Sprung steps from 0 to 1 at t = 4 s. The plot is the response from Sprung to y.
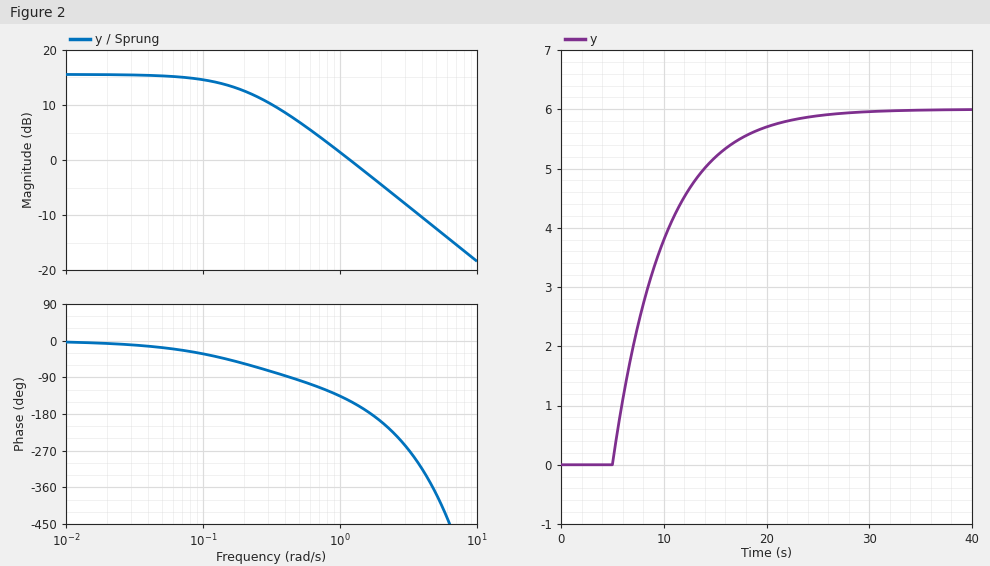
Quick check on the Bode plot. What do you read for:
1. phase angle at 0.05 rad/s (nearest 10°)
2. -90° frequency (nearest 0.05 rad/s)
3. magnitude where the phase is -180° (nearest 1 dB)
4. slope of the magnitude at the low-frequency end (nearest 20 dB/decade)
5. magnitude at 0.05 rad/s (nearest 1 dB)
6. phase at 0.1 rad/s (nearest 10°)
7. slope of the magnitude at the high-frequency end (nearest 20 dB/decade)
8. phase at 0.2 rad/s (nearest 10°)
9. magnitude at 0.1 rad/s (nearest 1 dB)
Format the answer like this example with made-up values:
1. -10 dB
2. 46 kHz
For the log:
1. -20°
2. 0.45 rad/s
3. -3 dB
4. 0 dB/decade
5. 15 dB
6. -30°
7. -20 dB/decade
8. -60°
9. 15 dB
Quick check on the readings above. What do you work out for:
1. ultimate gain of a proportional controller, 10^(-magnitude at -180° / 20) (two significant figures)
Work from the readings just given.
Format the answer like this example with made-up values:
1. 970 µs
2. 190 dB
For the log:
1. 1.4
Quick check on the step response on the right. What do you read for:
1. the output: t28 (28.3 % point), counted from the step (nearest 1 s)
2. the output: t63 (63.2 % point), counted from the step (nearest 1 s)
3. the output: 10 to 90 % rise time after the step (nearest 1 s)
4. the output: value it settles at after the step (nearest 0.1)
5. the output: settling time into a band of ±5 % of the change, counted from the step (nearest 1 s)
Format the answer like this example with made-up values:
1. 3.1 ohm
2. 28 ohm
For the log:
1. 3 s
2. 6 s
3. 11 s
4. 6.0
5. 16 s
